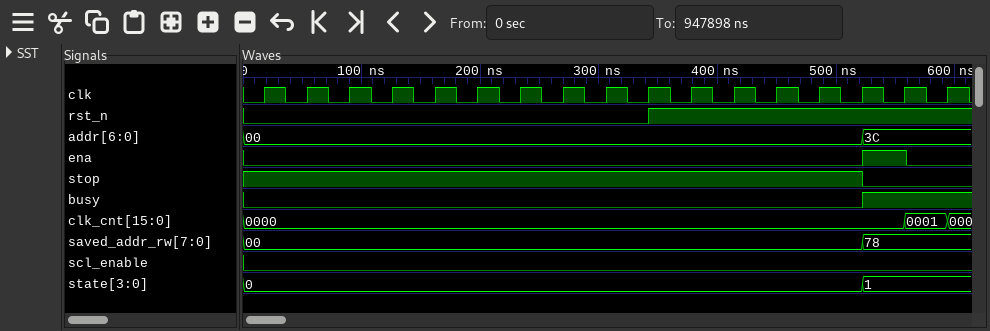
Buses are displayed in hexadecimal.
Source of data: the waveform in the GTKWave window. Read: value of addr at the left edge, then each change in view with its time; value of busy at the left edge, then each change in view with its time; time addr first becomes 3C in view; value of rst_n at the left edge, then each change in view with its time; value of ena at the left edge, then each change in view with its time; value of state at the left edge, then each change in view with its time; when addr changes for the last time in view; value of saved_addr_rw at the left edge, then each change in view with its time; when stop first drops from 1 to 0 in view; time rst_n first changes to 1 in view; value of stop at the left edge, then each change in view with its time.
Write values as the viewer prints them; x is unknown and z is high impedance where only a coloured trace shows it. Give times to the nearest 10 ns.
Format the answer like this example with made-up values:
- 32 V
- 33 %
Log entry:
- 00, 3C at 520 ns
- 0, 1 at 520 ns
- 520 ns
- 0, 1 at 340 ns
- 0, 1 at 520 ns, 0 at 560 ns
- 0, 1 at 520 ns
- 520 ns
- 00, 78 at 520 ns
- 520 ns
- 340 ns
- 1, 0 at 520 ns
